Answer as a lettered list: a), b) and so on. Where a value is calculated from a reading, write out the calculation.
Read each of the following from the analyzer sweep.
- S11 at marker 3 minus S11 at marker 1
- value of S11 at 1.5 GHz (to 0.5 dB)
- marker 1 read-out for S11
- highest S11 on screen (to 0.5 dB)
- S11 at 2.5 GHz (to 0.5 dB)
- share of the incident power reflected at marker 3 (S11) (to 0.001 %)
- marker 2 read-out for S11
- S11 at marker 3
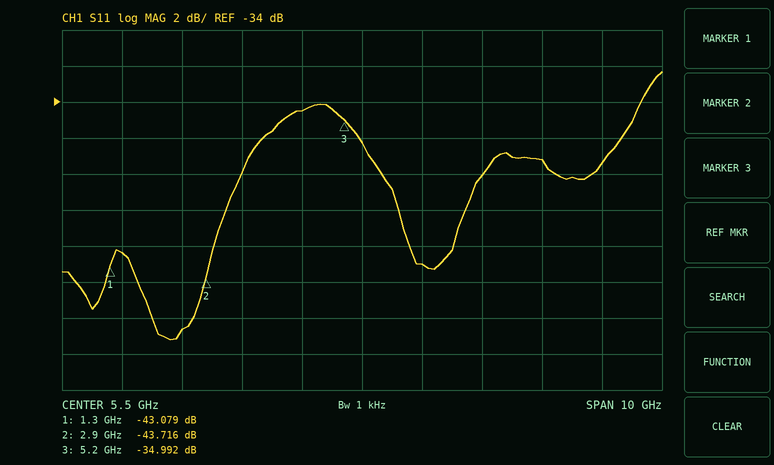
a) -34.992 − (-43.079) = 8.087 dB
b) -42.5 dB
c) -43.079 dB
d) -32.5 dB
e) -46.5 dB
f) 10^(-34.992/10) ≈ 0.032 %
g) -43.716 dB
h) -34.992 dB
